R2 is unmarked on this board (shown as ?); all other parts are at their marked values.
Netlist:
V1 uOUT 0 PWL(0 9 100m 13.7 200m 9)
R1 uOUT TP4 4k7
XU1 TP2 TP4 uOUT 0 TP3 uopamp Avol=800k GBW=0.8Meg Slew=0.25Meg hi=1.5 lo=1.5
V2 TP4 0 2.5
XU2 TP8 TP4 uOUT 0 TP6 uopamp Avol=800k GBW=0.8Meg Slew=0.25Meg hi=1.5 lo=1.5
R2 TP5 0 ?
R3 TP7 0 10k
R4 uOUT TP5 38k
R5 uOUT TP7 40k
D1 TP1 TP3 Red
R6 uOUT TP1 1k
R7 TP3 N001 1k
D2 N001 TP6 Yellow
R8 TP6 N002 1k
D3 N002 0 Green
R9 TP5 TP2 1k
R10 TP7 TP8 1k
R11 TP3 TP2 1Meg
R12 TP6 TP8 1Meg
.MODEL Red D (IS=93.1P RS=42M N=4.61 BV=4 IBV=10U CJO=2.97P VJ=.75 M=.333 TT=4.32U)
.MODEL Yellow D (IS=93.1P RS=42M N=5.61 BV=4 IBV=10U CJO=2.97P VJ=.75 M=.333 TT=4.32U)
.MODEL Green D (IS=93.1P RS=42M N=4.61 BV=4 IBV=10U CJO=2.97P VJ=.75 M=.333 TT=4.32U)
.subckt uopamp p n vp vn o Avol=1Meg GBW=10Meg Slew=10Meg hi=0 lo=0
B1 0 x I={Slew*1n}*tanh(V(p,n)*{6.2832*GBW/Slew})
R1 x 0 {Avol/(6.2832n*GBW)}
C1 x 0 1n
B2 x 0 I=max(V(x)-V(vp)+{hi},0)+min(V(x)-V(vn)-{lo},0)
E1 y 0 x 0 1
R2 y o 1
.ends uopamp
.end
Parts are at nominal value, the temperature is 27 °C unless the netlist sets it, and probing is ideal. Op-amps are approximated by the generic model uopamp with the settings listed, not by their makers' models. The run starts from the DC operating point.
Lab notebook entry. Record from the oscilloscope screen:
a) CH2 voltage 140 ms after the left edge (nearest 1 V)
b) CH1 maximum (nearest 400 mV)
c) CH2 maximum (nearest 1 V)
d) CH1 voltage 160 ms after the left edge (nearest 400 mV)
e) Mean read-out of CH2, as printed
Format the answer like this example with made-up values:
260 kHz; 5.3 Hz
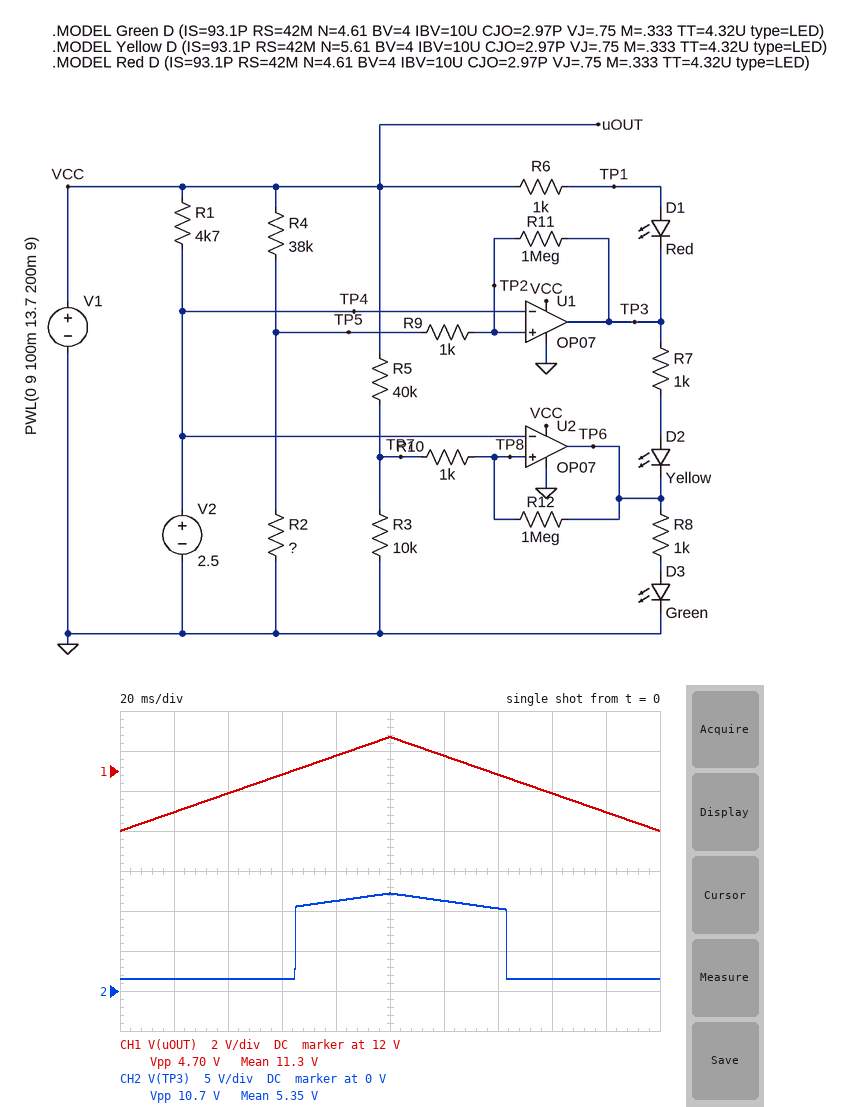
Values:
10 V; 13.6 V; 12 V; 10.8 V; 5.35 V
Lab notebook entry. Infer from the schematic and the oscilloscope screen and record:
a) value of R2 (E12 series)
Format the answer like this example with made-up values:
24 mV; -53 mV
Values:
10 kΩ
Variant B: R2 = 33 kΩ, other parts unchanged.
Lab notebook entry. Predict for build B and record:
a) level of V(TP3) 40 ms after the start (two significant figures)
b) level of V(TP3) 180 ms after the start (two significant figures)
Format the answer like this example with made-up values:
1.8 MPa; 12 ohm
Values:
9.4 V; 8.4 V
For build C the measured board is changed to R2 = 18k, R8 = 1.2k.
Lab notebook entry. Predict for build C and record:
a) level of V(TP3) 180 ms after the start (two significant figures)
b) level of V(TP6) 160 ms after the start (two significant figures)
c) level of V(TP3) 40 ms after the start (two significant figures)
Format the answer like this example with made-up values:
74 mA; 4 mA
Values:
8.4 V; 1.5 V; 9.4 V
